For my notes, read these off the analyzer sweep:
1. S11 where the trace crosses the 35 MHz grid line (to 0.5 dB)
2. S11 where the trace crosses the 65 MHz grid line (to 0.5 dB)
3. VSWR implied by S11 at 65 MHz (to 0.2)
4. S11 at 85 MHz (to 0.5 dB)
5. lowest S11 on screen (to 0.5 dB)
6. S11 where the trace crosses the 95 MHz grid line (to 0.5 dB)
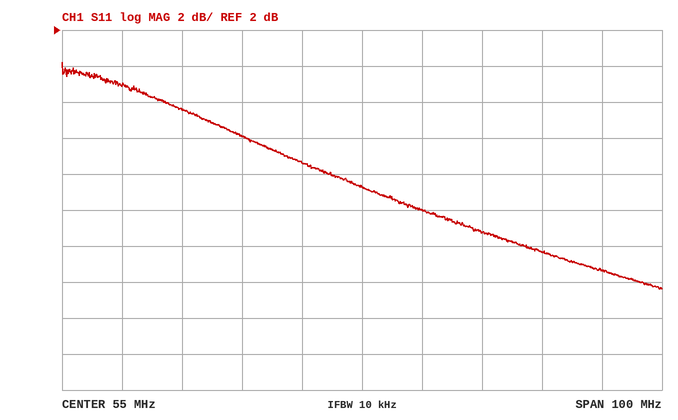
-4.0 dB
-8.0 dB
2.4
-10.5 dB
-12.5 dB
-11.5 dB
